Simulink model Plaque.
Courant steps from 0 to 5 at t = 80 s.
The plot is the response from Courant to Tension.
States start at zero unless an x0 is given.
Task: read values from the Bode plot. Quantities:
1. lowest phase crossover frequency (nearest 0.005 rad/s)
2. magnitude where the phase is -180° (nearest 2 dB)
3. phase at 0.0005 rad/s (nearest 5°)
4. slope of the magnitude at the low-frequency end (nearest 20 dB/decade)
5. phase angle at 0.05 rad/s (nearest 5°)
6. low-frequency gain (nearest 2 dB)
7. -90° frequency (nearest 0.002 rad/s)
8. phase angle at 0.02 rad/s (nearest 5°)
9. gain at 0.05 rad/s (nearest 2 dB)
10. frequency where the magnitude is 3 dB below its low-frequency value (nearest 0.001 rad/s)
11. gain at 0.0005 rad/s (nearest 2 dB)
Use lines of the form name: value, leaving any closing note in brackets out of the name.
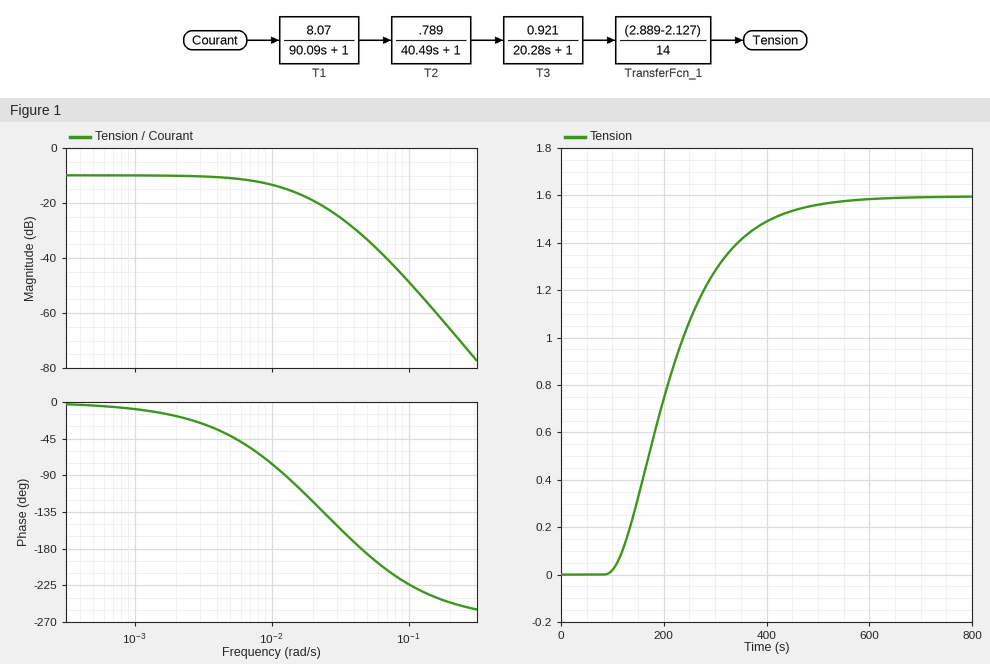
lowest phase crossover frequency: 0.045 rad/s
magnitude where the phase is -180°: -32 dB
phase at 0.0005 rad/s: -5°
slope of the magnitude at the low-frequency end: 0 dB/decade
phase angle at 0.05 rad/s: -185°
low-frequency gain: -10 dB
-90° frequency: 0.012 rad/s
phase angle at 0.02 rad/s: -120°
gain at 0.05 rad/s: -34 dB
frequency where the magnitude is 3 dB below its low-frequency value: 0.009 rad/s
gain at 0.0005 rad/s: -10 dB
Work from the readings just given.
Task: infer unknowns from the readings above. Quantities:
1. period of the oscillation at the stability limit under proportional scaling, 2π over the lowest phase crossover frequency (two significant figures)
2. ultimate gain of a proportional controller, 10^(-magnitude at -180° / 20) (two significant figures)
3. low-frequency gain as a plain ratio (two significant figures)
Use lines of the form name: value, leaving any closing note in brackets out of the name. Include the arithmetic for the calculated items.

period of the oscillation at the stability limit under proportional scaling, 2π over the lowest phase crossover frequency: 2π / 0.045 = 140 s
ultimate gain of a proportional controller, 10^(-magnitude at -180° / 20): 10^(32 / 20) = 40
low-frequency gain as a plain ratio: 10^(-10 / 20) = 0.32
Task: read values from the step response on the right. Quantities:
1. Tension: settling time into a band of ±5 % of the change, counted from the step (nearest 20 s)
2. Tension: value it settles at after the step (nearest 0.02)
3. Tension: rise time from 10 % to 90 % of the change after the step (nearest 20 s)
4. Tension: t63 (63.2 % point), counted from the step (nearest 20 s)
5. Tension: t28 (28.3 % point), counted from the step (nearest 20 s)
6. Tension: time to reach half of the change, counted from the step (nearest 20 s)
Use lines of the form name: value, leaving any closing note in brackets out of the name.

Tension: settling time into a band of ±5 % of the change, counted from the step: 340 s
Tension: value it settles at after the step: 1.60
Tension: rise time from 10 % to 90 % of the change after the step: 240 s
Tension: t63 (63.2 % point), counted from the step: 160 s
Tension: t28 (28.3 % point), counted from the step: 80 s
Tension: time to reach half of the change, counted from the step: 120 s
